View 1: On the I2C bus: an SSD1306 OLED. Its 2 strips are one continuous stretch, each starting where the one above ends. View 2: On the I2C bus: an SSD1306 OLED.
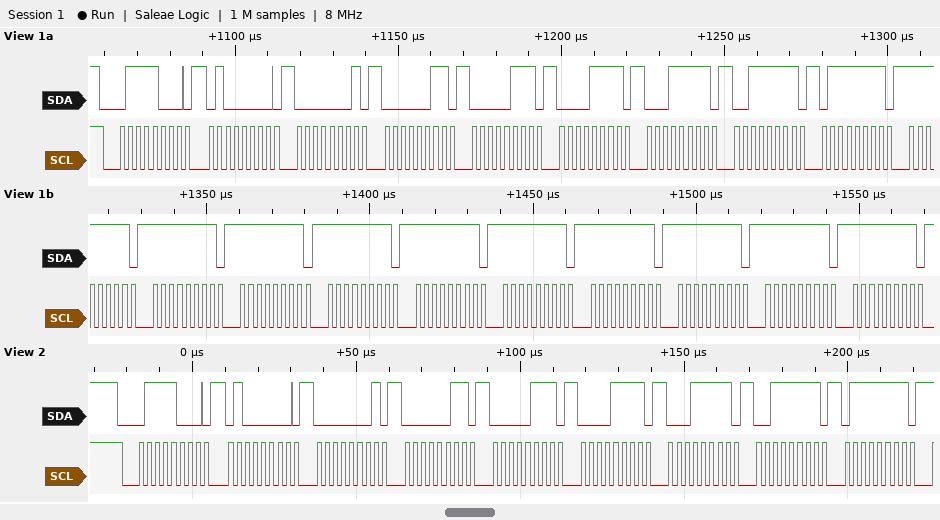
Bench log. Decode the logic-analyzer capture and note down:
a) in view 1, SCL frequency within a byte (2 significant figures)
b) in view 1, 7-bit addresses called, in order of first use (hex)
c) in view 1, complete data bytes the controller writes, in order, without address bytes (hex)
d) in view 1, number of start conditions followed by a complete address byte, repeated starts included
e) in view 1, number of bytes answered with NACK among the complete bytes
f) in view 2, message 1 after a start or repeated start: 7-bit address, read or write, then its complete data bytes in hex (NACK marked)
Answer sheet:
400 kHz
0x3C
40 01 03 07 0F 1F 3F 7F FF FF FF FF FF FF FF FF FF FF
1
0
0x3C write: 40 01 03 07 0F 1F 3F 7F
